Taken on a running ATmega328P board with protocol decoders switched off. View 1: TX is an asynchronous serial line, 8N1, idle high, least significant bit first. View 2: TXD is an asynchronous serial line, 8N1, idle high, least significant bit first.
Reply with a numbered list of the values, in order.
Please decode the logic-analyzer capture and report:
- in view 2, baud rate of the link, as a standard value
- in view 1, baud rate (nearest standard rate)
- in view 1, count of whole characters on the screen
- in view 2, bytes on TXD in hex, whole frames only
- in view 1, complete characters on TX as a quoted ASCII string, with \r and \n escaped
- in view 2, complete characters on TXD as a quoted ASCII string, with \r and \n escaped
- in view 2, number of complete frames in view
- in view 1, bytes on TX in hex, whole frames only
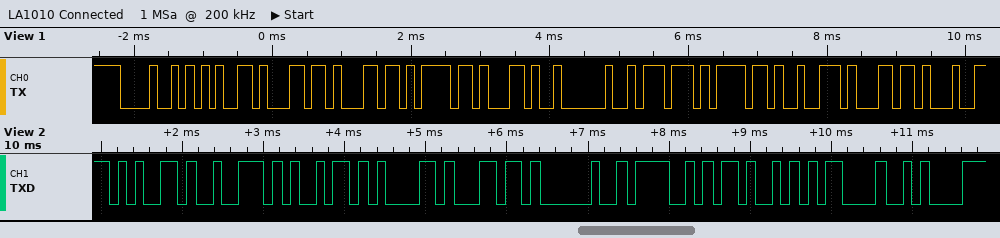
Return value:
1. 9600 baud
2. 9600 baud
3. 11
4. 65 72 69 61 6C 20 4F 4B 0D 0A
5. "Hello, worl"
6. "erial OK\r\n"
7. 10
8. 48 65 6C 6C 6F 2C 20 77 6F 72 6C
